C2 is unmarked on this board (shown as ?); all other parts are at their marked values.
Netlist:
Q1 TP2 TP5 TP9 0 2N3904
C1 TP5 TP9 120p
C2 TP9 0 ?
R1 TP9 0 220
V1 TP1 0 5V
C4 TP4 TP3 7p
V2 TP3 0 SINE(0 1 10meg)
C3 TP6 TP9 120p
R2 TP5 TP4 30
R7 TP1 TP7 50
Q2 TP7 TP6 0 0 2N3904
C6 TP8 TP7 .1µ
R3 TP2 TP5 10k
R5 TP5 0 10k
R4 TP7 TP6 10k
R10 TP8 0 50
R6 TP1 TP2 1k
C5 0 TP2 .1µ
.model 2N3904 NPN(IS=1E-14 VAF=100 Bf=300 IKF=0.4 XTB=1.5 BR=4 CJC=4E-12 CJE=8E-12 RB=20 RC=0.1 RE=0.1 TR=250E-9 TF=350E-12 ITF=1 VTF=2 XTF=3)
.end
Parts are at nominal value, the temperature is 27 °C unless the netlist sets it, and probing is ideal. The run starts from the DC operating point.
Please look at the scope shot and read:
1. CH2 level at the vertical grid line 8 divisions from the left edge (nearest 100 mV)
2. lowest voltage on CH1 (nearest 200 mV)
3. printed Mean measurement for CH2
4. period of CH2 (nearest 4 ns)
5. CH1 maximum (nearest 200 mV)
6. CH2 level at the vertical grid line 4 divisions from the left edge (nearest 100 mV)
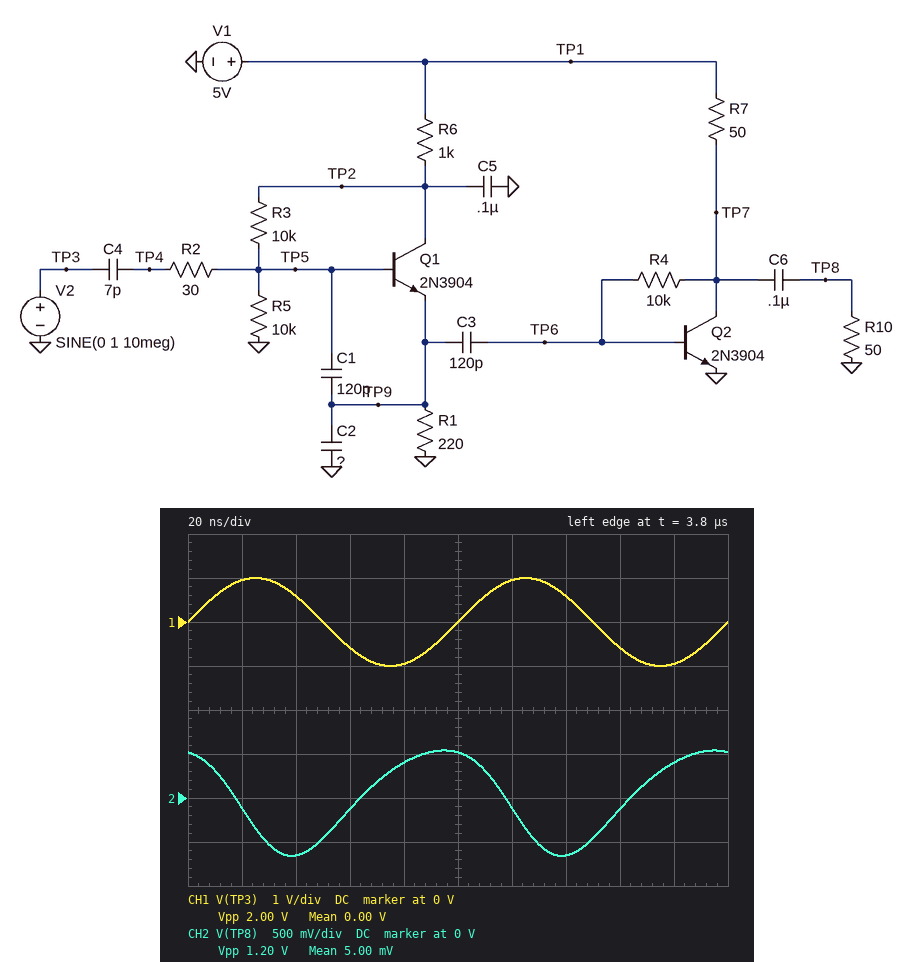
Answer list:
-100 mV
-1.0 V
5.00 mV
100 ns
1.0 V
400 mV
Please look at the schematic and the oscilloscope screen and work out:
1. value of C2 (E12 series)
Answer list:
330 pF
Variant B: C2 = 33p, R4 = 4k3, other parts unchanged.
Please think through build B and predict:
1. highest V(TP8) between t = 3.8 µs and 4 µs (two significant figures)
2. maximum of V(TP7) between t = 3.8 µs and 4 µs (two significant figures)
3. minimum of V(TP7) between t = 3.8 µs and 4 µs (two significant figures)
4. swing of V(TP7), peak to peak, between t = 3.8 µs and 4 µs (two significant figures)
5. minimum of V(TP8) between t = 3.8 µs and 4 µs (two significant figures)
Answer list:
1.2 V
3.0 V
460 mV
2.5 V
-1.4 V
